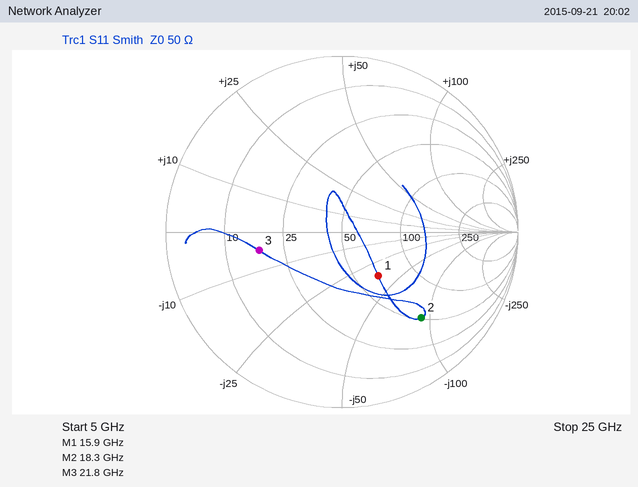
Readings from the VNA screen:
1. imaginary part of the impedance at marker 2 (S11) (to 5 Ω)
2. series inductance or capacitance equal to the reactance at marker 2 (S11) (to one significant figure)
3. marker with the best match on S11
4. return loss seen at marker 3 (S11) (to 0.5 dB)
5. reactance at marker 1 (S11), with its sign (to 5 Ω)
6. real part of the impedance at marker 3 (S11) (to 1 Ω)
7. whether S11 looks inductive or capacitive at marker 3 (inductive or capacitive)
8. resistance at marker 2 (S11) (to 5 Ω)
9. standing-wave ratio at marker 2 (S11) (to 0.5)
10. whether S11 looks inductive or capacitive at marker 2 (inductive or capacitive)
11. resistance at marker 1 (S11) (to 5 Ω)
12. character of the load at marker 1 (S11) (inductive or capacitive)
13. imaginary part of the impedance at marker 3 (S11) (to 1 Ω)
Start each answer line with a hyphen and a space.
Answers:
- -90 Ω
- 100 fF
- marker 1
- 6.5 dB
- -35 Ω
- 18 Ω
- capacitive
- 50 Ω
- 5.0
- capacitive
- 65 Ω
- capacitive
- -5 Ω
